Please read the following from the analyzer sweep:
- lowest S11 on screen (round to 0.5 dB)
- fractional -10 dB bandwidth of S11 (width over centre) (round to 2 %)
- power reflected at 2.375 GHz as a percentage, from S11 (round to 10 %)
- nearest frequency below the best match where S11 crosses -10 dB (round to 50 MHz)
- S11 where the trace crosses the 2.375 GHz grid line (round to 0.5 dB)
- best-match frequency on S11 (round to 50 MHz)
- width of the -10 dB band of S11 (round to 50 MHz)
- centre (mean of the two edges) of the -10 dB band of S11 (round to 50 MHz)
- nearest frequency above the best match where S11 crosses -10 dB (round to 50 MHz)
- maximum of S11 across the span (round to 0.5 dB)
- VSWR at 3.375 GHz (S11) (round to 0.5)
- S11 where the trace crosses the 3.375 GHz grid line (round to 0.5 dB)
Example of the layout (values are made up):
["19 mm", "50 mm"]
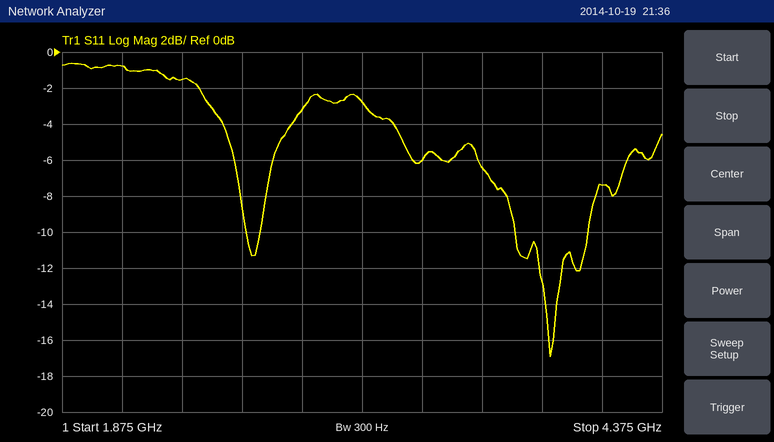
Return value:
["-17.0 dB", "8 %", "70 %", "3.75 GHz", "-1.5 dB", "3.90 GHz", "300 MHz", "3.90 GHz", "4.05 GHz", "-0.5 dB", "3.0", "-6.0 dB"]
